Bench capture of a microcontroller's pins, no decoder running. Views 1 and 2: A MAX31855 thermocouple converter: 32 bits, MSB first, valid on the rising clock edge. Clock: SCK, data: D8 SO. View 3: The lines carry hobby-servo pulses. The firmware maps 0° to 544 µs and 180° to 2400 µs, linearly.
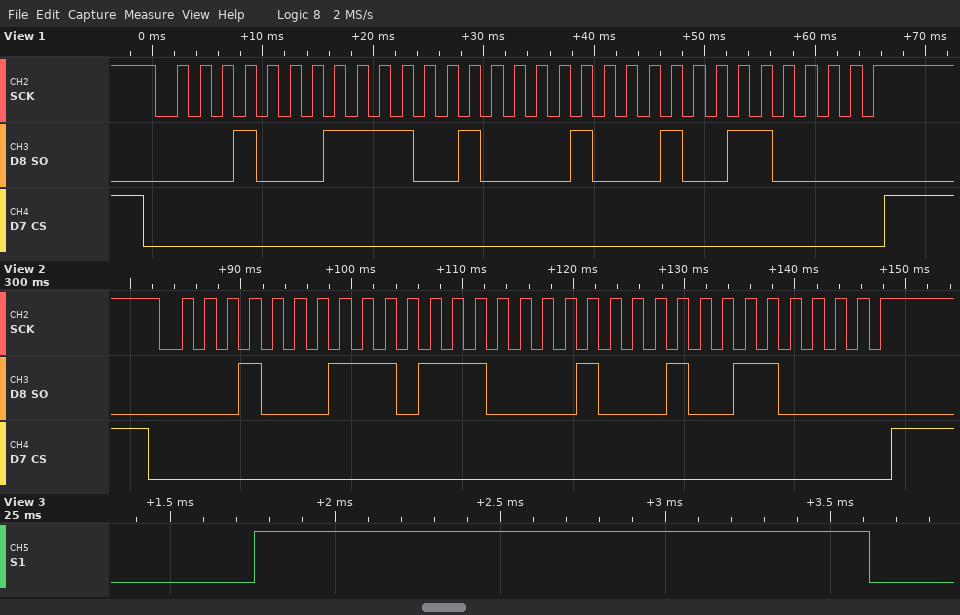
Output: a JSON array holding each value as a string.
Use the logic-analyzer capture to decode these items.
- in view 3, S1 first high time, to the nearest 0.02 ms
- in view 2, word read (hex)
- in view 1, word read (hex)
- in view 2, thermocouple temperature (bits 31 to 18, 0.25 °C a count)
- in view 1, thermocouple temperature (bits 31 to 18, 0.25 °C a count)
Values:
["1.86 ms", "0x11DC2260", "0x11E42260", "285.75 °C", "286.25 °C"]
